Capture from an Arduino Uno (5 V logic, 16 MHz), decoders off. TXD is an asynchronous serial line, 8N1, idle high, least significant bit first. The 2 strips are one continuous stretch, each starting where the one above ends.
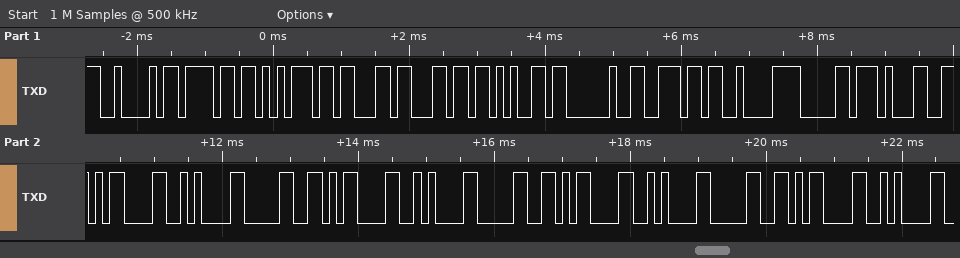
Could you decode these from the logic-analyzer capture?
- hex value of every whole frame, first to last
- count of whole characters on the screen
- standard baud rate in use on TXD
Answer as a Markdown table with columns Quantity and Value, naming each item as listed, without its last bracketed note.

| Quantity | Value |
|---|---|
| hex value of every whole frame, first to last | 42 6F 75 63 6C 65 20 6E C2 B0 31 0D 0A 30 0D 0A 30 0D 0A 30 0D 0A |
| count of whole characters on the screen | 22 |
| standard baud rate in use on TXD | 9600 baud |
